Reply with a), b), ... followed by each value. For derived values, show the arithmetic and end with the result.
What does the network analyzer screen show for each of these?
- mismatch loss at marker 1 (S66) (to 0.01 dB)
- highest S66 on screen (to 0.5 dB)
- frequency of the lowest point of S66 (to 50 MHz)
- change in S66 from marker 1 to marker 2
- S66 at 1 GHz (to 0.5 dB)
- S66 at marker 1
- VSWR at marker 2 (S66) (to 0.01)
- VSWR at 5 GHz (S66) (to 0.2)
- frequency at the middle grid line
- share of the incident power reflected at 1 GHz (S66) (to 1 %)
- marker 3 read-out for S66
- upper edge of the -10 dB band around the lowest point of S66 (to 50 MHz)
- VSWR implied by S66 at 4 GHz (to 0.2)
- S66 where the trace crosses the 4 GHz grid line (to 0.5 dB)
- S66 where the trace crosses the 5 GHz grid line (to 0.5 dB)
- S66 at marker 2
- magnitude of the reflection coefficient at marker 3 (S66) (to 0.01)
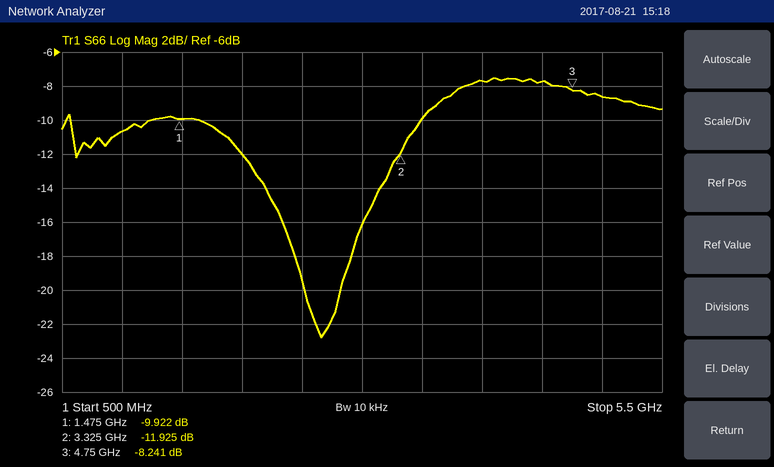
a) −10 log10(1 − 10^(-9.922/10)) ≈ 0.47 dB
b) -7.5 dB
c) 2.65 GHz
d) -11.925 − (-9.922) = -2.003 dB
e) -10.5 dB
f) -9.922 dB
g) (1 + 0.2534)/(1 − 0.2534) ≈ 1.68
h) |Γ| = 10^(-8.5/20) = 0.3758; VSWR = (1 + 0.3758)/(1 − 0.3758) ≈ 2.2
i) 3 GHz
j) 10^(-10.5/10) ≈ 9 %
k) -8.241 dB
l) 3.50 GHz
m) |Γ| = 10^(-7.5/20) = 0.4217; VSWR = (1 + 0.4217)/(1 − 0.4217) ≈ 2.46, so 2.4 to the nearest 0.2
n) -7.5 dB
o) -8.5 dB
p) -11.925 dB
q) 10^(-8.241/20) ≈ 0.39
